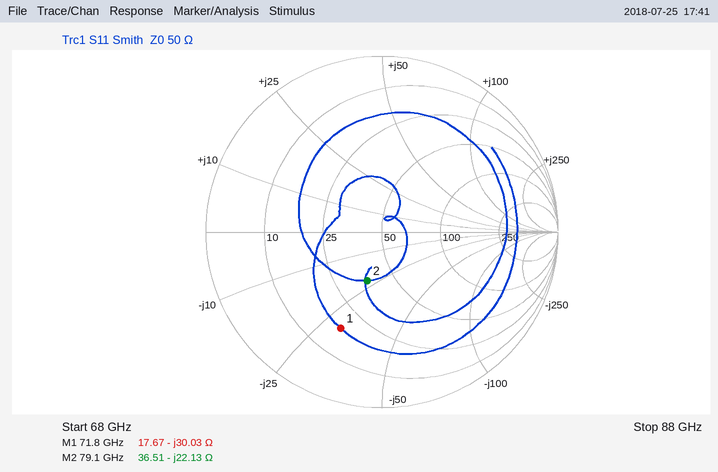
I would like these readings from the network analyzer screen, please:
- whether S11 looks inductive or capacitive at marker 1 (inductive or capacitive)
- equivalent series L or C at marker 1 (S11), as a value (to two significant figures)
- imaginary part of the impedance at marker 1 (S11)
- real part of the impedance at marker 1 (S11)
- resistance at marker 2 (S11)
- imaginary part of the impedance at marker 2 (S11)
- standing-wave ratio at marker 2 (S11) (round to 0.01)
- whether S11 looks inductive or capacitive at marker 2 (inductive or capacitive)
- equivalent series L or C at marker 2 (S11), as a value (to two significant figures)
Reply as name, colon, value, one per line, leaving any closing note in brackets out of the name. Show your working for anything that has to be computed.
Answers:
whether S11 looks inductive or capacitive at marker 1: capacitive
equivalent series L or C at marker 1 (S11), as a value: C = 1/(2π × 71.8 GHz × 30.03 Ω) ≈ 74 fF
imaginary part of the impedance at marker 1: -30.03 Ω
real part of the impedance at marker 1: 17.67 Ω
resistance at marker 2: 36.51 Ω
imaginary part of the impedance at marker 2: -22.13 Ω
standing-wave ratio at marker 2 (S11): 1.82
whether S11 looks inductive or capacitive at marker 2: capacitive
equivalent series L or C at marker 2 (S11), as a value: C = 1/(2π × 79.1 GHz × 22.13 Ω) ≈ 91 fF
